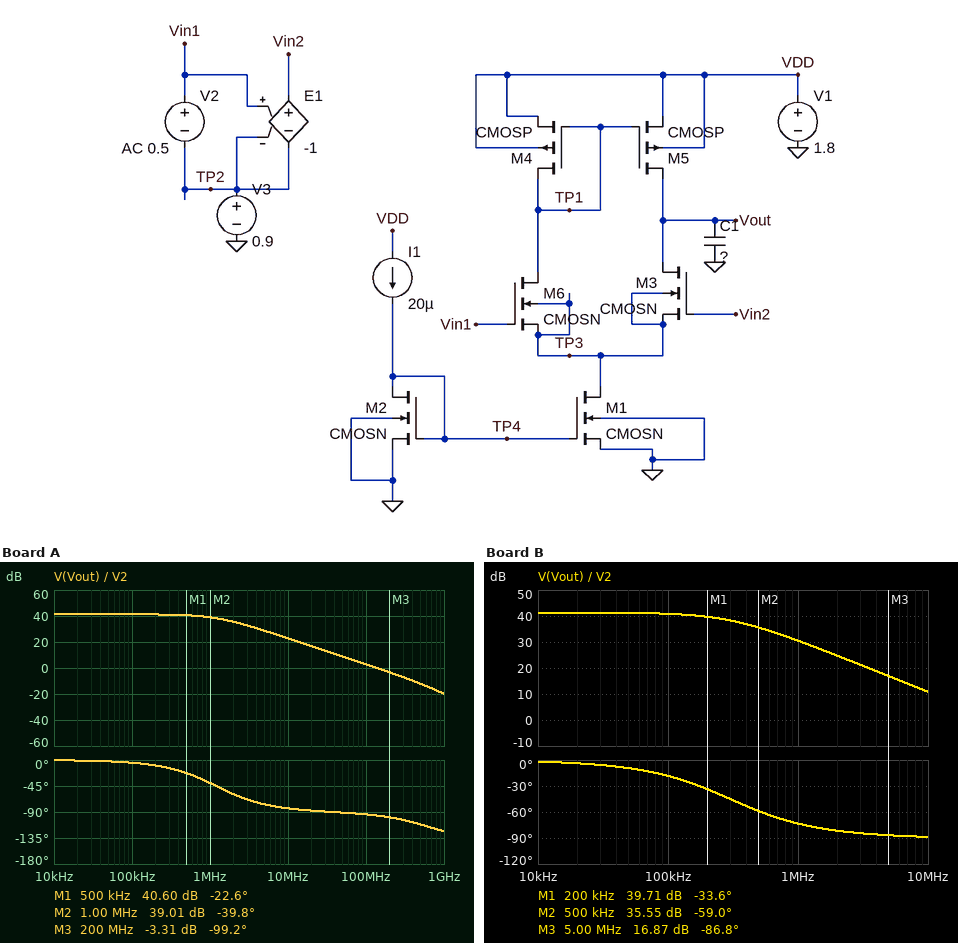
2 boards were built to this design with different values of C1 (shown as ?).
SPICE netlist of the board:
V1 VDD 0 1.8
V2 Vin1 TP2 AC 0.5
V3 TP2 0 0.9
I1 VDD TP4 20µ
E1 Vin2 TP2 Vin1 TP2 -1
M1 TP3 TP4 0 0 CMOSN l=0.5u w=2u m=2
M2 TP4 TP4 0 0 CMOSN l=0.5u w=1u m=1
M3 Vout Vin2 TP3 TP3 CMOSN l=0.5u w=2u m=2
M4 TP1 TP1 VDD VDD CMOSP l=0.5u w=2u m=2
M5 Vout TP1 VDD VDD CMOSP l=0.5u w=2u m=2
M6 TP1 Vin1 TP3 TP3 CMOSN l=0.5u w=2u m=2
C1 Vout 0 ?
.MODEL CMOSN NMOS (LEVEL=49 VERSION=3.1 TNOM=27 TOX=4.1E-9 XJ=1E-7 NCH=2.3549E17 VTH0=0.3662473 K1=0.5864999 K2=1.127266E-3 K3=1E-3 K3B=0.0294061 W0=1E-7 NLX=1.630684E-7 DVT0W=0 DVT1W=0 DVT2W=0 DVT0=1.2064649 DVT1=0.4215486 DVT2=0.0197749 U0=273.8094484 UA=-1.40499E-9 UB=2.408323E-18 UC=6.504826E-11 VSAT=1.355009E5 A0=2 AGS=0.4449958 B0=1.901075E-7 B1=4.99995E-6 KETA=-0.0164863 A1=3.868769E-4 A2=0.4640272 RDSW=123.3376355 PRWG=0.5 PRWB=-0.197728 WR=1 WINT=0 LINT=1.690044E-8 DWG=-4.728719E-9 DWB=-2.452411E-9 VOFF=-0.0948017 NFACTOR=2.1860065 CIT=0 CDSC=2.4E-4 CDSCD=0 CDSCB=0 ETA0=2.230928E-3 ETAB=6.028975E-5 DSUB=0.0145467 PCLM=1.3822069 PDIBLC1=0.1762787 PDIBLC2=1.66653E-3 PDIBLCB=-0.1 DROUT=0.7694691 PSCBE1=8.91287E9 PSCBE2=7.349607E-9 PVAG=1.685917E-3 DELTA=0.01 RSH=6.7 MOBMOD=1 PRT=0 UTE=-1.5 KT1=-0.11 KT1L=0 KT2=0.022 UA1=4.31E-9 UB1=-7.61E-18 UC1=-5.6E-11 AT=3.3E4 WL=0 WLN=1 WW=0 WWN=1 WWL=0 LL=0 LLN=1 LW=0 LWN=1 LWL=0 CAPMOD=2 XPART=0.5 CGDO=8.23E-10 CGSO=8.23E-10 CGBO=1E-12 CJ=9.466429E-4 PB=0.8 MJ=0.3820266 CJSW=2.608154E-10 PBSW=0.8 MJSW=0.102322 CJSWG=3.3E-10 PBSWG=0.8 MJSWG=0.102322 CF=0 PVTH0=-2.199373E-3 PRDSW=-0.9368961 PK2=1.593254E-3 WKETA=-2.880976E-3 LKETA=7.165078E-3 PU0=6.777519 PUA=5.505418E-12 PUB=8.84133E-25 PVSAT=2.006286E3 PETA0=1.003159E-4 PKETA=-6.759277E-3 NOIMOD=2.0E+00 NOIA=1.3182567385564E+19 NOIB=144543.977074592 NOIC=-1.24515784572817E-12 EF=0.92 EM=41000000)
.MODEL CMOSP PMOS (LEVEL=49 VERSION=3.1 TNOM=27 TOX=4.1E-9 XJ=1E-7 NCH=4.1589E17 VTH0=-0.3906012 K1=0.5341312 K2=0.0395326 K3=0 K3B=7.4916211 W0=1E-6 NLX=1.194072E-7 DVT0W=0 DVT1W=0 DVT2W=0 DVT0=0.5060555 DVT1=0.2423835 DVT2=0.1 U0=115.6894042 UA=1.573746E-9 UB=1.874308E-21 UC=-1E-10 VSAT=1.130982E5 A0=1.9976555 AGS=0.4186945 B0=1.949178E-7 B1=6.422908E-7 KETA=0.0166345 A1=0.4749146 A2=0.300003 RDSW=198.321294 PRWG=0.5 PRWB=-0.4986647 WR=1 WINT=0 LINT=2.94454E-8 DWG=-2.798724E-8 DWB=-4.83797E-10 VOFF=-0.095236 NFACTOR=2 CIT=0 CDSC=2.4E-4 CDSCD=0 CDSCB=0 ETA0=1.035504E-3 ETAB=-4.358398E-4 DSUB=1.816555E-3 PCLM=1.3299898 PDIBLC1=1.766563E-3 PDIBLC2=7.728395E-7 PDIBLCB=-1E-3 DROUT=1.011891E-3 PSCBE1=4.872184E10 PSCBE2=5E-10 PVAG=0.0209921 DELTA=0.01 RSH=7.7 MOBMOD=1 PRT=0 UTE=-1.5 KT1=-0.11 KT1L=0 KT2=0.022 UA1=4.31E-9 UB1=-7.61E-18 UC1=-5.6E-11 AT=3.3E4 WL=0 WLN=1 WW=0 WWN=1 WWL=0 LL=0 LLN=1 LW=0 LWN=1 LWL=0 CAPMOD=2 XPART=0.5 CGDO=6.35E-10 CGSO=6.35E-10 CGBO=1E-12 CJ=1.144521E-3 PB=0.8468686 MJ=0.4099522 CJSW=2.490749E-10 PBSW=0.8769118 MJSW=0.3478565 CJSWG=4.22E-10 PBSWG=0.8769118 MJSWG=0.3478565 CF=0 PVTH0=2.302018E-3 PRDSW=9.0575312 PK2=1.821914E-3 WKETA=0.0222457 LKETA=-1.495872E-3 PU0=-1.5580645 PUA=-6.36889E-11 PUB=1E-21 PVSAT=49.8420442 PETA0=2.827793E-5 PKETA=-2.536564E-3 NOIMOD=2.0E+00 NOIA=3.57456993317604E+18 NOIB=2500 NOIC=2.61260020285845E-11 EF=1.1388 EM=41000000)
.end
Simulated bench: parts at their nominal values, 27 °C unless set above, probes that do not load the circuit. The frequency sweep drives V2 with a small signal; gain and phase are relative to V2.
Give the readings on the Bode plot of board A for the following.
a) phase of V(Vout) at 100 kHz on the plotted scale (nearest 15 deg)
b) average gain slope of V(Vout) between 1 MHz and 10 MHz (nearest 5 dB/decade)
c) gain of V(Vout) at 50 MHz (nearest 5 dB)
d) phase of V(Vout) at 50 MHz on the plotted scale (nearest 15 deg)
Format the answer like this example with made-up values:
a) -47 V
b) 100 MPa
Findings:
a) 0 deg
b) -15 dB/decade
c) 10 dB
d) -90 deg
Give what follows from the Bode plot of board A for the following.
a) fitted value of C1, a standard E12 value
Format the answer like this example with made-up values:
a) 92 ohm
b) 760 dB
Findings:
a) 820 fF
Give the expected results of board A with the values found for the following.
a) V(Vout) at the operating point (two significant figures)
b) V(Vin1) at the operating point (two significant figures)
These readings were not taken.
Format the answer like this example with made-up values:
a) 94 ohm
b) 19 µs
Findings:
a) 980 mV
b) 900 mV
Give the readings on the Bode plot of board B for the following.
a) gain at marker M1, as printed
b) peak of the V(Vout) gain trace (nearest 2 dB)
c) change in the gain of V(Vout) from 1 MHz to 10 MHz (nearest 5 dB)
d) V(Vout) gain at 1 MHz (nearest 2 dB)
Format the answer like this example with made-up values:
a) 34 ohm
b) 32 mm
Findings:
a) 39.71 dB
b) 42 dB
c) -20 dB
d) 30 dB
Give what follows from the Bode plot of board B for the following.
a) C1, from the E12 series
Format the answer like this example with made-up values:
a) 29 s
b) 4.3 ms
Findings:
a) 3.3 pF
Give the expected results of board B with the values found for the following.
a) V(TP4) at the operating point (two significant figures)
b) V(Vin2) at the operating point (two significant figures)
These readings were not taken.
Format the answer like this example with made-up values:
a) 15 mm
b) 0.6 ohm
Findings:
a) 720 mV
b) 900 mV
